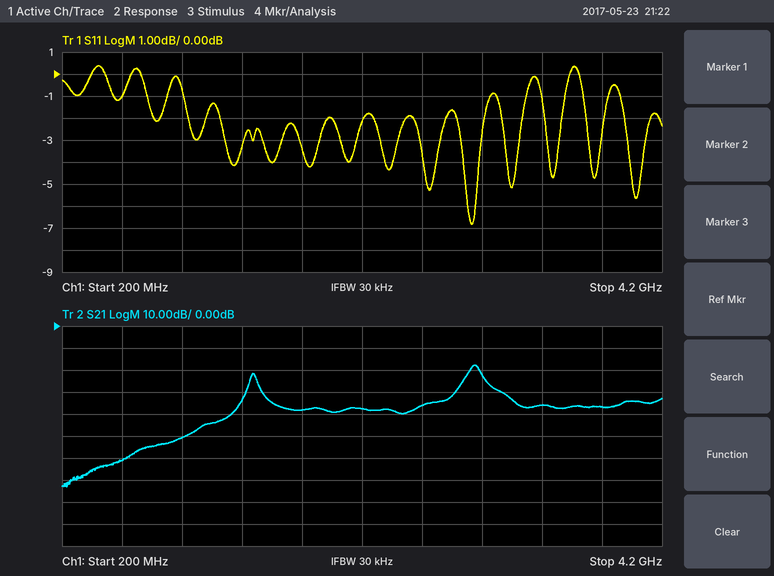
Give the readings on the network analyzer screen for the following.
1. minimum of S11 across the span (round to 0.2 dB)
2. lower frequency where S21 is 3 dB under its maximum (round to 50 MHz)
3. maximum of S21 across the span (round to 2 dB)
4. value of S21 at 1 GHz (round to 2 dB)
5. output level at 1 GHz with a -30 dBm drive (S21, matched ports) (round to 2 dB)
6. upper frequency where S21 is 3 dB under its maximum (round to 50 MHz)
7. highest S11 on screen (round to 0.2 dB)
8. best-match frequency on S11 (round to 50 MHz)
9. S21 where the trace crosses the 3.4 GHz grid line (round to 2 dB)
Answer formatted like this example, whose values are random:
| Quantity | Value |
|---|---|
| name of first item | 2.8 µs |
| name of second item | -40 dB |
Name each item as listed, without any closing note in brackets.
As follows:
| Quantity | Value |
|---|---|
| minimum of S11 across the span | -6.8 dB |
| lower frequency where S21 is 3 dB under its maximum | 2.90 GHz |
| maximum of S21 across the span | -18 dB |
| value of S21 at 1 GHz | -50 dB |
| output level at 1 GHz with a -30 dBm drive (S21, matched ports) | -80 dBm |
| upper frequency where S21 is 3 dB under its maximum | 3.00 GHz |
| highest S11 on screen | 0.4 dB |
| best-match frequency on S11 | 2.95 GHz |
| S21 where the trace crosses the 3.4 GHz grid line | -36 dB |
